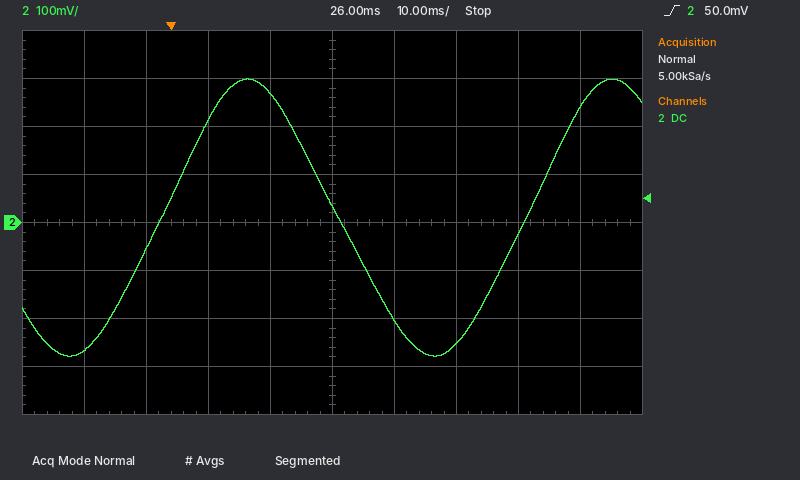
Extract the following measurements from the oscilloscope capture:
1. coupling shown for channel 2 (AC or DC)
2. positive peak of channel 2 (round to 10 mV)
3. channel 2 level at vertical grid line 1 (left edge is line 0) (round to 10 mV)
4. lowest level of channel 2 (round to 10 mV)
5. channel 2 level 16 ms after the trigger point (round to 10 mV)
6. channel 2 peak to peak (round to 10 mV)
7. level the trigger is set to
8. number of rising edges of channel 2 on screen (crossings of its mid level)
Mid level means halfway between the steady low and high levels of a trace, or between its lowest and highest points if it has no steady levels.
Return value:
DC
300 mV
-270 mV
-280 mV
270 mV
580 mV
50.0 mV
2
